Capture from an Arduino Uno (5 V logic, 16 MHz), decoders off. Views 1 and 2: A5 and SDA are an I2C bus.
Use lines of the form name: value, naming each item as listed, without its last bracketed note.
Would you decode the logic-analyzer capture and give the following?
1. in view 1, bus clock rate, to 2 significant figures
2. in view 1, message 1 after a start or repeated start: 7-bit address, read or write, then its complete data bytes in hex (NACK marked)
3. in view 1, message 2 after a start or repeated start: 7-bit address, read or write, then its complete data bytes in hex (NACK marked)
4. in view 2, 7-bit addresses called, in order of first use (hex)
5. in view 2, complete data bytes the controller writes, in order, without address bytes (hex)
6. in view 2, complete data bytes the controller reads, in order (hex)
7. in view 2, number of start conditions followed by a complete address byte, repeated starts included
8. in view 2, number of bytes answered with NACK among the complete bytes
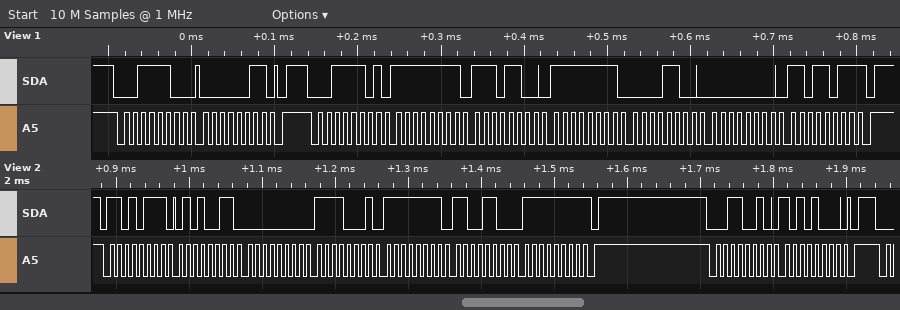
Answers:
in view 1, bus clock rate, to 2 significant figures: 100 kHz
in view 1, message 1 after a start or repeated start: 7-bit address, read or write, then its complete data bytes in hex: 0x1E write: 03
in view 1, message 2 after a start or repeated start: 7-bit address, read or write, then its complete data bytes in hex: 0x1E read: FF EC FF 0C 00 DB NACK
in view 2, 7-bit addresses called, in order of first use: 0x6B 0x19
in view 2, complete data bytes the controller writes, in order, without address bytes: A8
in view 2, complete data bytes the controller reads, in order: 53 00 F1 FF CC FF
in view 2, number of start conditions followed by a complete address byte, repeated starts included: 2
in view 2, number of bytes answered with NACK among the complete bytes: 1
